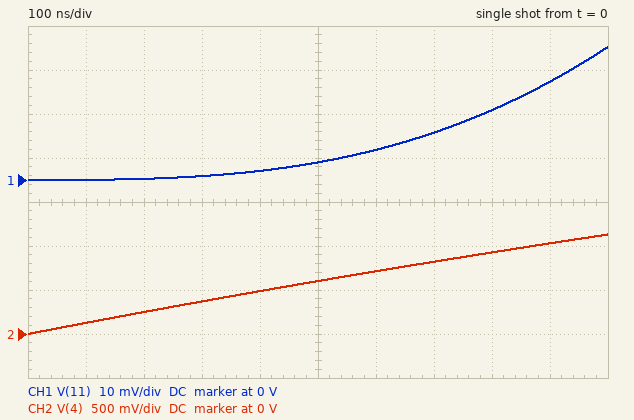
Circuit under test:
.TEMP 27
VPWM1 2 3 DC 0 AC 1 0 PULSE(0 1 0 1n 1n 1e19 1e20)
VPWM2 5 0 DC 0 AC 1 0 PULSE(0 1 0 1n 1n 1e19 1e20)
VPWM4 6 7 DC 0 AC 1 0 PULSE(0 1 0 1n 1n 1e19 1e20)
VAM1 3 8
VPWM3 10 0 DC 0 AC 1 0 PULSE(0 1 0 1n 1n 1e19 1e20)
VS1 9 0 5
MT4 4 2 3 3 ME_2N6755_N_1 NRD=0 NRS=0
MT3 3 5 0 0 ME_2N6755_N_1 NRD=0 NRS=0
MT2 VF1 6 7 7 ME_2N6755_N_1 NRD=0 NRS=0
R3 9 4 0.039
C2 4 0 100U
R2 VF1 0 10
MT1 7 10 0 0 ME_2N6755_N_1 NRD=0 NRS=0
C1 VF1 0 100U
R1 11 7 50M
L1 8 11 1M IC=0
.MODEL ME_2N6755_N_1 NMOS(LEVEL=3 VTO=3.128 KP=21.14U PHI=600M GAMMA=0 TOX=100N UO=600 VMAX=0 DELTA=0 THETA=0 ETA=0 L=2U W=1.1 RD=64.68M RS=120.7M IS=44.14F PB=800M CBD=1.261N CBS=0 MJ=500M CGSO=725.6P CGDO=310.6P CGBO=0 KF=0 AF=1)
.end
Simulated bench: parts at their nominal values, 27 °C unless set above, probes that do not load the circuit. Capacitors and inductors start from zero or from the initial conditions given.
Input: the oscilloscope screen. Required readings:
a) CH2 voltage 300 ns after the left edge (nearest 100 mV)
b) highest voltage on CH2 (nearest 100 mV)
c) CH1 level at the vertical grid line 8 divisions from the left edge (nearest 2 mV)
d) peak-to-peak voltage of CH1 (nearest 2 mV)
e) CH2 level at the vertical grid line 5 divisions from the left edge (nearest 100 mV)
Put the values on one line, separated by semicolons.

400 mV; 1.1 V; 16 mV; 30 mV; 600 mV
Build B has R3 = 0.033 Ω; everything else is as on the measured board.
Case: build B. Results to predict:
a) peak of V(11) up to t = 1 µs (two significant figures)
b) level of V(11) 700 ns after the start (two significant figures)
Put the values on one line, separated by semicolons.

35 mV; 13 mV
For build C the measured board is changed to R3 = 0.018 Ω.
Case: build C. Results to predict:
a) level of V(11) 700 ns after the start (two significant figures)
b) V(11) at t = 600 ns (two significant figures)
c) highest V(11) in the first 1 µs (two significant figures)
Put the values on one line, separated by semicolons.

22 mV; 14 mV; 61 mV
